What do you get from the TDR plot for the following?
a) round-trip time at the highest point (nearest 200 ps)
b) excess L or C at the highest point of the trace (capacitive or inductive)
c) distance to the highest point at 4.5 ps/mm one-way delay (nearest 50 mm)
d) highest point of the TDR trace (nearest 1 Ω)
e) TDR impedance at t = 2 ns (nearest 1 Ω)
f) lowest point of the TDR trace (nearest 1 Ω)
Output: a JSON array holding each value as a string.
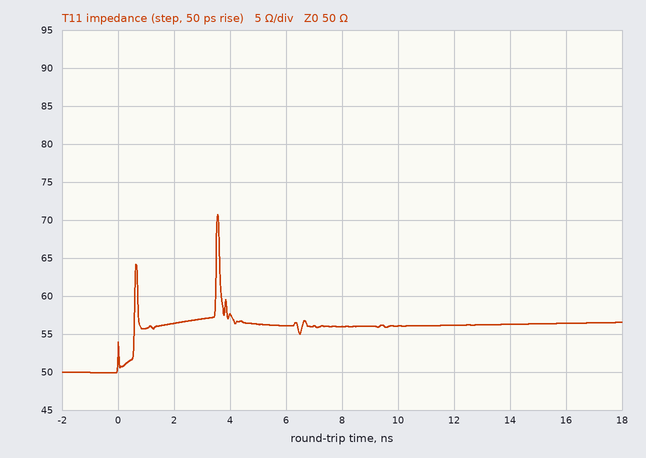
["3.6 ns", "inductive", "400 mm", "71 Ω", "56 Ω", "50 Ω"]
